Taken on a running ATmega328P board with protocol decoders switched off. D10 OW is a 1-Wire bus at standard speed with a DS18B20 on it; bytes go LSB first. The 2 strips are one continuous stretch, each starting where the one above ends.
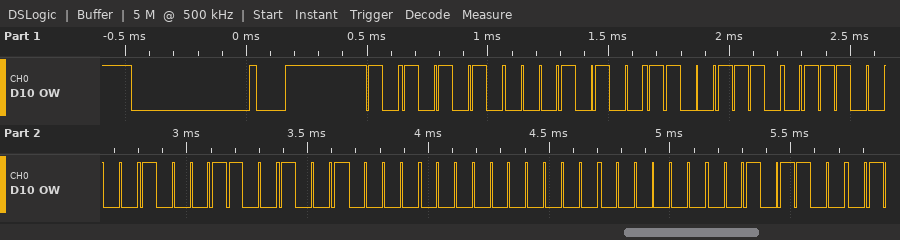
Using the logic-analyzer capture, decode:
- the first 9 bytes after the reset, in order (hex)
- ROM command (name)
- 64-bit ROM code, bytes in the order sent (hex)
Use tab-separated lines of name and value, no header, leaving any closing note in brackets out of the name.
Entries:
the first 9 bytes after the reset, in order	55 28 73 0E 31 09 00 00 34
ROM command	Match ROM
64-bit ROM code, bytes in the order sent	28 73 0E 31 09 00 00 34
